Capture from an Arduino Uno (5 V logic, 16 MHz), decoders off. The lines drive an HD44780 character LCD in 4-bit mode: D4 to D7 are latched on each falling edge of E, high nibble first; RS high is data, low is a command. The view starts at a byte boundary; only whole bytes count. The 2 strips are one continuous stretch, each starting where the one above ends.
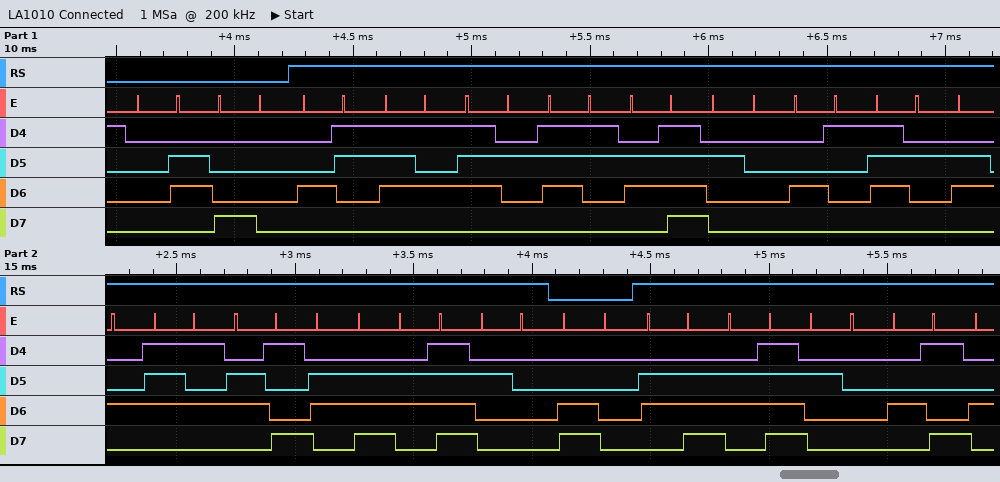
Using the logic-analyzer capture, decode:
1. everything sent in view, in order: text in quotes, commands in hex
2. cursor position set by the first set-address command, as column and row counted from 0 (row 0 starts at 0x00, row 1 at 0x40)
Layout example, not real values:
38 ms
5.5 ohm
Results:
0x06 0x80 "Curso Arduino " 0xC0 "no I"
column 0, row 0
